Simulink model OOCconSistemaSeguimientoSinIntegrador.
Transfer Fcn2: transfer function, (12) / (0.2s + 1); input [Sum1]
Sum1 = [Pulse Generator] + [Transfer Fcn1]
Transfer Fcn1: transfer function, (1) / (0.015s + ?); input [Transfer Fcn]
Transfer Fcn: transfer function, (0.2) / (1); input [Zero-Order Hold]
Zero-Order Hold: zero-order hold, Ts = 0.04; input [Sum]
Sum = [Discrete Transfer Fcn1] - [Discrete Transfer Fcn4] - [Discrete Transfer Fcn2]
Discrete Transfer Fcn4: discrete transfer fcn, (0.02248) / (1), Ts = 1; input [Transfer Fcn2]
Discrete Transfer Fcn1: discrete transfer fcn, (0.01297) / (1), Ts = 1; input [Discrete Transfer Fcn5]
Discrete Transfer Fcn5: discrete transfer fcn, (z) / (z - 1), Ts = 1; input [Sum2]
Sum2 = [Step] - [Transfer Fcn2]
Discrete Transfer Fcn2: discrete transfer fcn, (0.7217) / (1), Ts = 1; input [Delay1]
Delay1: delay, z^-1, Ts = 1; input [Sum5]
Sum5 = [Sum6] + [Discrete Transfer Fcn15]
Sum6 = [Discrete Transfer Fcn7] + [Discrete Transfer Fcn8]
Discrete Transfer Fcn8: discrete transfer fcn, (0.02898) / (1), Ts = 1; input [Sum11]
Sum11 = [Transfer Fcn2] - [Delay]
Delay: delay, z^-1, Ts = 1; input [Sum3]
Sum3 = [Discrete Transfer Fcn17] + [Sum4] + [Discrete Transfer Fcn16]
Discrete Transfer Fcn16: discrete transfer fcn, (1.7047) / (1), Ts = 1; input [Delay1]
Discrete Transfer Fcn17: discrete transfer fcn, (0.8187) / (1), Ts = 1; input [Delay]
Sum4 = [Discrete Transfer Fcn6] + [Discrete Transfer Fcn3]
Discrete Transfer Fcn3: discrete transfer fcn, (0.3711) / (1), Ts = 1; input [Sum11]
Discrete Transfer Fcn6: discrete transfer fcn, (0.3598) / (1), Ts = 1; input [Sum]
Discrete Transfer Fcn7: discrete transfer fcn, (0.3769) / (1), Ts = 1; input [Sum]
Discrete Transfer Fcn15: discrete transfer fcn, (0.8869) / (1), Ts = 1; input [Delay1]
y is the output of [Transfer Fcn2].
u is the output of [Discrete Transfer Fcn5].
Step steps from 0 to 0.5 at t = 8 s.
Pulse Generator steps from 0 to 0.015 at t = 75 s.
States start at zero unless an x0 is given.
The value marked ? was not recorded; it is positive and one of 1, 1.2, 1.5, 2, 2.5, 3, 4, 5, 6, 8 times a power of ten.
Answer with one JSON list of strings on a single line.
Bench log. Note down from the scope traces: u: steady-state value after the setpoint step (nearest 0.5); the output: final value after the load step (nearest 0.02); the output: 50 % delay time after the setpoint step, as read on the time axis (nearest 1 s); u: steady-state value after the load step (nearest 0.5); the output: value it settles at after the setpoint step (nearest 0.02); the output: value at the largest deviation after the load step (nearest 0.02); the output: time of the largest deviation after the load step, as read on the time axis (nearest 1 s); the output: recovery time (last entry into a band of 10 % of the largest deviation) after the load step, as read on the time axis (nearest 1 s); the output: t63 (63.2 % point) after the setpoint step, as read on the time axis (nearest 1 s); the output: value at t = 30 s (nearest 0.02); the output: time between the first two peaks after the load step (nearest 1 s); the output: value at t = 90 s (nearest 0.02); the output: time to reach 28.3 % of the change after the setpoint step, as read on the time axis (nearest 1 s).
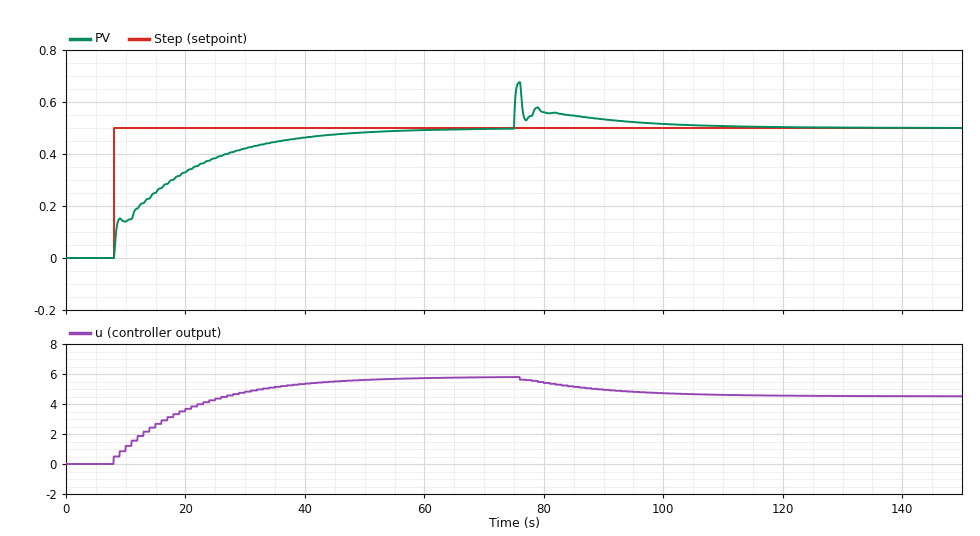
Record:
["6.0", "0.50", "15 s", "4.5", "0.50", "0.68", "76 s", "98 s", "19 s", "0.42", "3 s", "0.54", "9 s"]
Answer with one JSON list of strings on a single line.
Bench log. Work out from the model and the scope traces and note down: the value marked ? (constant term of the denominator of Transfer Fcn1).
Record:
["0.1"]
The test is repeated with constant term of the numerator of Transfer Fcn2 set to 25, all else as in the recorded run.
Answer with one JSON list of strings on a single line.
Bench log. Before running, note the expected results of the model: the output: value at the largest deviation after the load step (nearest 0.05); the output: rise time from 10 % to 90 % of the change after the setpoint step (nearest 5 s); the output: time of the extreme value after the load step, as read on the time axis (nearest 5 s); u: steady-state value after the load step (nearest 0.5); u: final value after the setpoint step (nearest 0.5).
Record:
["0.90", "20 s", "80 s", "2.5", "4.0"]
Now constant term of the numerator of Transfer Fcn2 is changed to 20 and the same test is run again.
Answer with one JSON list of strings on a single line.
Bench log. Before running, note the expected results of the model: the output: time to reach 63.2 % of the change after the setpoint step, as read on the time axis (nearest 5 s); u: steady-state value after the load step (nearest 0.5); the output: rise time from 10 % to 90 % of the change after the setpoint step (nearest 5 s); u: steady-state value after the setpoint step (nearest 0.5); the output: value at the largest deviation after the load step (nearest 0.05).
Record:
["15 s", "3.0", "20 s", "4.5", "0.80"]
